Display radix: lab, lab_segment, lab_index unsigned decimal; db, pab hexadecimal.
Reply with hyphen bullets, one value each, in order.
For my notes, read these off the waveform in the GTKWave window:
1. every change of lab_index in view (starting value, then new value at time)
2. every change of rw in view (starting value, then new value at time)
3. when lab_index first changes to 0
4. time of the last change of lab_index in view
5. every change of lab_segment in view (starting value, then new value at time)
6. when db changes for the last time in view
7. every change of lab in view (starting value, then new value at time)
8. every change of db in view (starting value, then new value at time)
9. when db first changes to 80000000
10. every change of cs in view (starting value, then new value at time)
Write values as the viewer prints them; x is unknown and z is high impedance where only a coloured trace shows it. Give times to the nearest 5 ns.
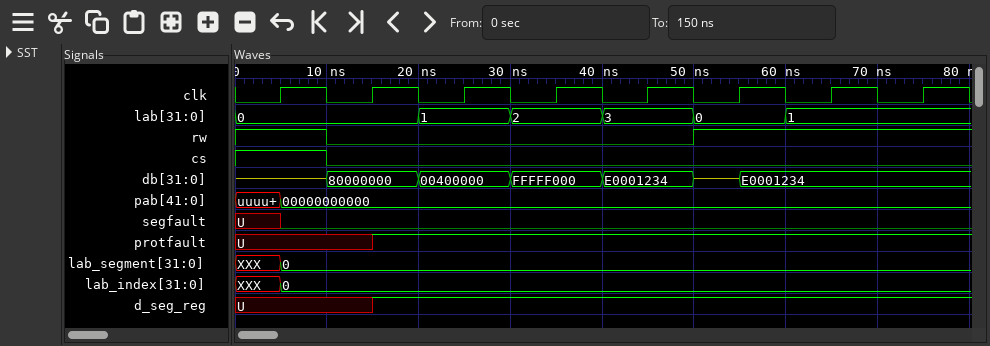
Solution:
- XXX, 0 at 5 ns
- 1, 0 at 10 ns, 1 at 50 ns
- 5 ns
- 5 ns
- XXX, 0 at 5 ns
- 55 ns
- 0, 1 at 20 ns, 2 at 30 ns, 3 at 40 ns, 0 at 50 ns, 1 at 60 ns
- z, 80000000 at 10 ns, 00400000 at 20 ns, FFFFF000 at 30 ns, E0001234 at 40 ns, z at 50 ns, E0001234 at 55 ns
- 10 ns
- 1, 0 at 10 ns
